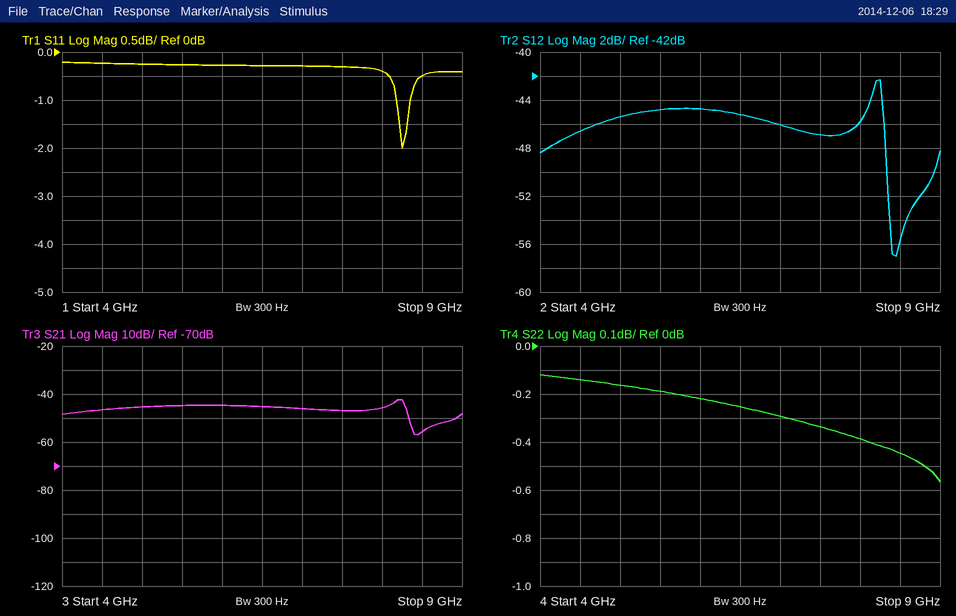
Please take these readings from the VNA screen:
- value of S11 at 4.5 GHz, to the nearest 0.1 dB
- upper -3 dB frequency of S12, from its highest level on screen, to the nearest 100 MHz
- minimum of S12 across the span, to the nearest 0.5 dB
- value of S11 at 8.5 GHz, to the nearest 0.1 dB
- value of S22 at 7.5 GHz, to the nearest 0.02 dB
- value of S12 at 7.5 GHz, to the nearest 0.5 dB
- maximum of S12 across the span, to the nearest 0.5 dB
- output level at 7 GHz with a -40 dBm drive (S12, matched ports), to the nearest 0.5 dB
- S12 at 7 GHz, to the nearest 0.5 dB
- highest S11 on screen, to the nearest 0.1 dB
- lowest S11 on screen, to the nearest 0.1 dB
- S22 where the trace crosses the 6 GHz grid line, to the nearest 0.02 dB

-0.2 dB
8.3 GHz
-57.0 dB
-0.5 dB
-0.34 dB
-47.0 dB
-42.5 dB
-86.0 dBm
-46.0 dB
-0.2 dB
-2.0 dB
-0.22 dB
